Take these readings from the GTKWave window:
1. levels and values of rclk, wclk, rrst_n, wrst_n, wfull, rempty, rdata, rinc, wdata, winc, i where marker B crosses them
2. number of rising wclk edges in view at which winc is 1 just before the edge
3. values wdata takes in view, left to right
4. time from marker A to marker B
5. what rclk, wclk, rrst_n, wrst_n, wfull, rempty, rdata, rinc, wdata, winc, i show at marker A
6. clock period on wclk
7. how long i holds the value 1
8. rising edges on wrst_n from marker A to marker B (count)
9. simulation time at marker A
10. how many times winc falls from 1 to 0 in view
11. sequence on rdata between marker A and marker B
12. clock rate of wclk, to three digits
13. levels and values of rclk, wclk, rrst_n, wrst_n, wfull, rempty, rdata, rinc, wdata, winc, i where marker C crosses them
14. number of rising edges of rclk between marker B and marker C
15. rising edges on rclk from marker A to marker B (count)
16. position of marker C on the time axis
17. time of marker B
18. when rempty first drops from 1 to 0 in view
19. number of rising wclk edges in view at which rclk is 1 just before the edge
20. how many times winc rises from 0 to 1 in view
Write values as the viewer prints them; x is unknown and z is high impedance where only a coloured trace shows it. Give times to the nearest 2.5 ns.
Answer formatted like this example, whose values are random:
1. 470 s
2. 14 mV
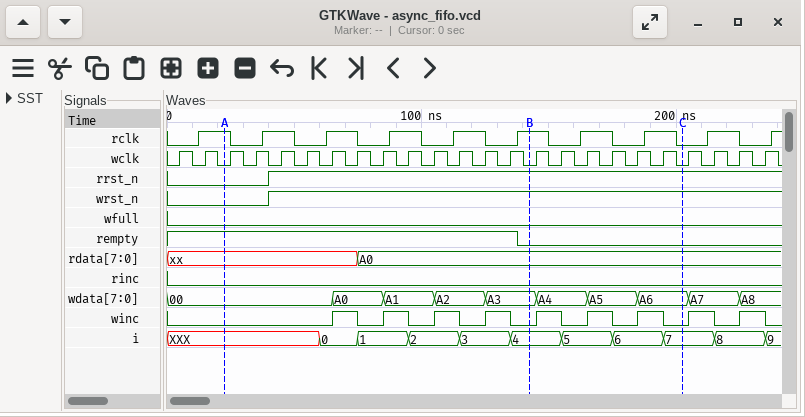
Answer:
1. rclk=1, wclk=0, rrst_n=1, wrst_n=1, wfull=0, rempty=0, rdata=A0, rinc=0, wdata=A3, winc=0, i=4
2. 9
3. 00, A0, A1, A2, A3, A4, A5, A6, A7, A8
4. 120 ns
5. rclk=1, wclk=0, rrst_n=0, wrst_n=0, wfull=0, rempty=1, rdata=xx, rinc=0, wdata=00, winc=0, i=XXX
6. 10 ns
7. 20 ns
8. 1
9. 22.5 ns
10. 9
11. xx, A0
12. 100 MHz
13. rclk=0, wclk=0, rrst_n=1, wrst_n=1, wfull=0, rempty=0, rdata=A0, rinc=0, wdata=A6, winc=0, i=7
14. 2
15. 5
16. 202.5 ns
17. 142.5 ns
18. 137.5 ns
19. 14
20. 9
